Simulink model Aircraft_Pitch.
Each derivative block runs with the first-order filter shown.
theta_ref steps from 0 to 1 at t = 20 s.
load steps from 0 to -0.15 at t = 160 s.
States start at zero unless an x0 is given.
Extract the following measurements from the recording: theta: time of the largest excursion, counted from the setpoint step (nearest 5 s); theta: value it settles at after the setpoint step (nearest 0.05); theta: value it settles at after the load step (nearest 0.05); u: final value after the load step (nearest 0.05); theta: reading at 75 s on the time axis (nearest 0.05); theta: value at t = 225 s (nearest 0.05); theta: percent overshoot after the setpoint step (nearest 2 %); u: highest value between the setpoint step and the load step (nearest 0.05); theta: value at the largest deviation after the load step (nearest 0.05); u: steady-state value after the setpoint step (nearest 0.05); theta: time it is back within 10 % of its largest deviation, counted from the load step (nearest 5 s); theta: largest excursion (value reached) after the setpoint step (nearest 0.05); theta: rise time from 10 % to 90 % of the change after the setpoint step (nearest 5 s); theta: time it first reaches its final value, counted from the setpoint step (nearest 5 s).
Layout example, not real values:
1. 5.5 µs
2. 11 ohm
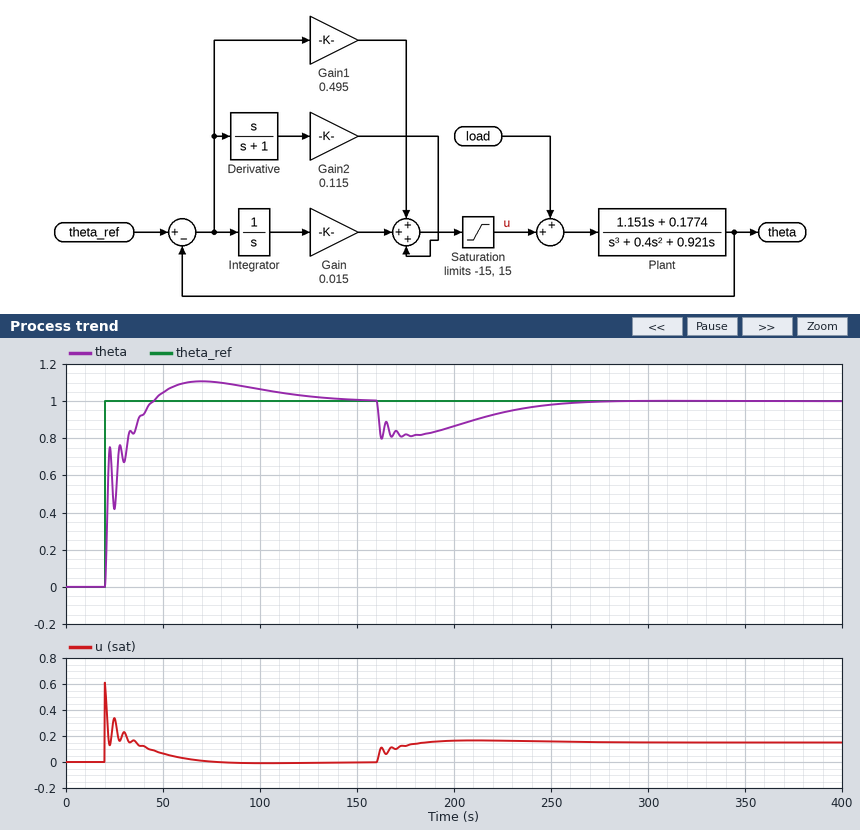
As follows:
1. 50 s
2. 1.00
3. 1.00
4. 0.15
5. 1.10
6. 0.95
7. 10 %
8. 0.60
9. 0.80
10. 0.00
11. 90 s
12. 1.10
13. 15 s
14. 25 s
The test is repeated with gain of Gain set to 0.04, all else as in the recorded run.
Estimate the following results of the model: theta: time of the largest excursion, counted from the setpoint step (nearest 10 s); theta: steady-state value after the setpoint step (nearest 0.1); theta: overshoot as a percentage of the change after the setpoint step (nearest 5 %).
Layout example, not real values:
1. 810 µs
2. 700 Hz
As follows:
1. 30 s
2. 1.0
3. 15 %
